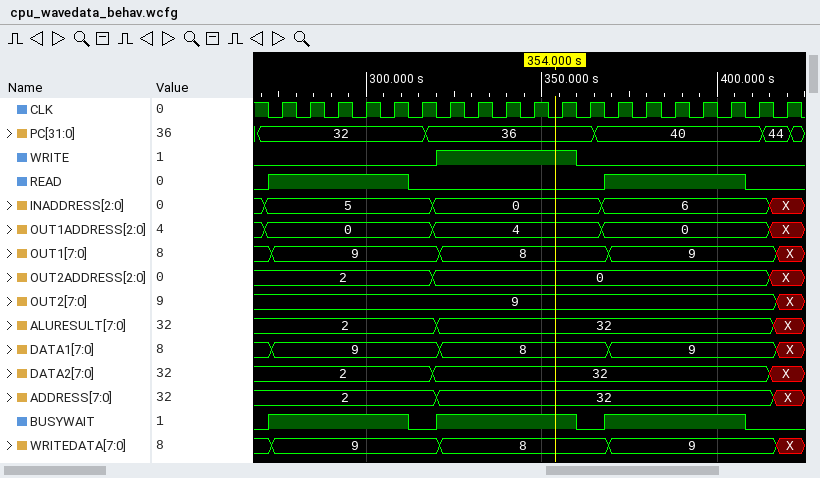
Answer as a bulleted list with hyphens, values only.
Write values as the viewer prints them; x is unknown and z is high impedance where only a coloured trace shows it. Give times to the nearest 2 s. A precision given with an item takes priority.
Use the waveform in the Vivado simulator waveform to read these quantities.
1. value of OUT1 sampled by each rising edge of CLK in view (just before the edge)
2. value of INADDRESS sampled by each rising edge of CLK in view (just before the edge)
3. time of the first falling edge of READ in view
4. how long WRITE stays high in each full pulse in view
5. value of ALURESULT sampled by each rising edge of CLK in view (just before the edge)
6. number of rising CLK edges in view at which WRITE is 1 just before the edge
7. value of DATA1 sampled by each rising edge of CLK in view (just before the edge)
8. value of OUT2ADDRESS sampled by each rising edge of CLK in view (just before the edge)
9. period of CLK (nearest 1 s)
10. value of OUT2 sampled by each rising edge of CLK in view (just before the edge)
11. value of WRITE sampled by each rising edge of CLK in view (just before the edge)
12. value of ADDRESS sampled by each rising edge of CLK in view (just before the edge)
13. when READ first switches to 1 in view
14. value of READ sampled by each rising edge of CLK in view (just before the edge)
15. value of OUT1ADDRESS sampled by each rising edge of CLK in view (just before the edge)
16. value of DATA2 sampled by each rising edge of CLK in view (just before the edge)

- 9, 9, 9, 9, 9, 9, 8, 8, 8, 8, 8, 8, 9, 9, 9, 9, 9, 9, X
- 5, 5, 5, 5, 5, 5, 0, 0, 0, 0, 0, 0, 6, 6, 6, 6, 6, 6, X
- 312 s
- 40 s
- 2, 2, 2, 2, 2, 2, 32, 32, 32, 32, 32, 32, 32, 32, 32, 32, 32, 32, X
- 5
- 9, 9, 9, 9, 9, 9, 8, 8, 8, 8, 8, 8, 9, 9, 9, 9, 9, 9, X
- 2, 2, 2, 2, 2, 2, 0, 0, 0, 0, 0, 0, 0, 0, 0, 0, 0, 0, X
- 8 s
- 9, 9, 9, 9, 9, 9, 9, 9, 9, 9, 9, 9, 9, 9, 9, 9, 9, 9, X
- 0 0 0 0 0 0 1 1 1 1 1 0 0 0 0 0 0 0 0
- 2, 2, 2, 2, 2, 2, 32, 32, 32, 32, 32, 32, 32, 32, 32, 32, 32, 32, X
- 272 s
- 1 1 1 1 1 0 0 0 0 0 0 0 1 1 1 1 1 0 0
- 0, 0, 0, 0, 0, 0, 4, 4, 4, 4, 4, 4, 0, 0, 0, 0, 0, 0, X
- 2, 2, 2, 2, 2, 2, 32, 32, 32, 32, 32, 32, 32, 32, 32, 32, 32, 32, X
